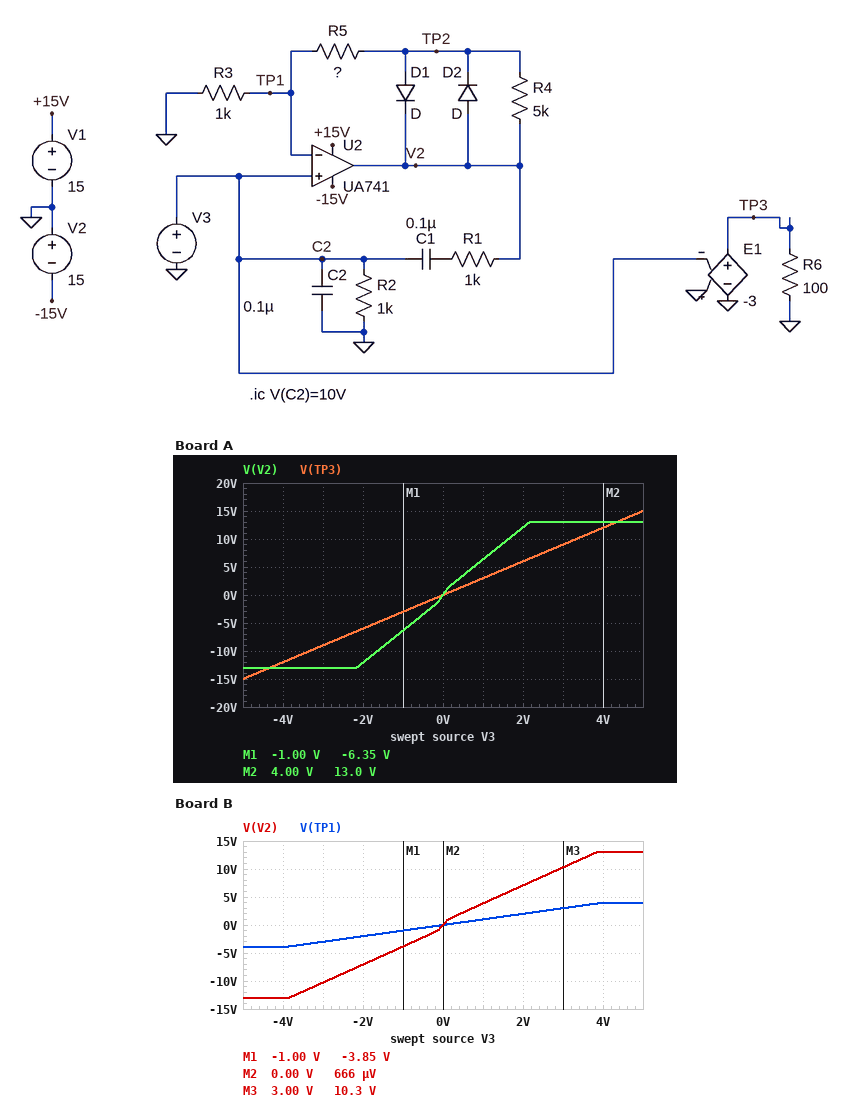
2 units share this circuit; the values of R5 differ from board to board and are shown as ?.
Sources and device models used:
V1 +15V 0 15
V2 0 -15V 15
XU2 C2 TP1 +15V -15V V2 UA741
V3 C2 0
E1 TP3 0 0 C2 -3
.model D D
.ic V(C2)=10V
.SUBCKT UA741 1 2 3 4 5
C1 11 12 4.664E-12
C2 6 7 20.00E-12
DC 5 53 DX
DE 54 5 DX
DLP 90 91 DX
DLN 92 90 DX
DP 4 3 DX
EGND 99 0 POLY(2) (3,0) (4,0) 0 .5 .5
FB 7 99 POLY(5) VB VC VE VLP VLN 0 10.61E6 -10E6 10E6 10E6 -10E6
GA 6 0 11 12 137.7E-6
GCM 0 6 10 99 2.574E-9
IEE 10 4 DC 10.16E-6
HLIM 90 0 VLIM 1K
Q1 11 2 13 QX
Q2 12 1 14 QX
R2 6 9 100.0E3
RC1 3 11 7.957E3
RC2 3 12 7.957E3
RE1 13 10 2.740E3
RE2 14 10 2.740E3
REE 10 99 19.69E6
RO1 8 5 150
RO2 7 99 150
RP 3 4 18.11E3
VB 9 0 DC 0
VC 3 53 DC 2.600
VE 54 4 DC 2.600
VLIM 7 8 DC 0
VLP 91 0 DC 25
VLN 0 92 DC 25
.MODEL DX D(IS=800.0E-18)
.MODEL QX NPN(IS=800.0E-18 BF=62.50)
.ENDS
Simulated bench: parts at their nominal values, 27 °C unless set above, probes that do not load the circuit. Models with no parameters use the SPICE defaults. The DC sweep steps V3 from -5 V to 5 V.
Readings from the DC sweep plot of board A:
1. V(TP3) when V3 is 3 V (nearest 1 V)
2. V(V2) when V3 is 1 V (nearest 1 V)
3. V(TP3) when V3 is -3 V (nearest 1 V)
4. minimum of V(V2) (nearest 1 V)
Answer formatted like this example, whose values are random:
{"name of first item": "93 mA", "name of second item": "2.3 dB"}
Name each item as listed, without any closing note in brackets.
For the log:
{"V(TP3) when V3 is 3 V": "9 V", "V(V2) when V3 is 1 V": "6 V", "V(TP3) when V3 is -3 V": "-9 V", "minimum of V(V2)": "-13 V"}
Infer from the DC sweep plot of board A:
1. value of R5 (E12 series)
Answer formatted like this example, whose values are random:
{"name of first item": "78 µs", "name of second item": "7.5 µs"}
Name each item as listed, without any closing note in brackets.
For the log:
{"value of R5": "4.7 kΩ"}
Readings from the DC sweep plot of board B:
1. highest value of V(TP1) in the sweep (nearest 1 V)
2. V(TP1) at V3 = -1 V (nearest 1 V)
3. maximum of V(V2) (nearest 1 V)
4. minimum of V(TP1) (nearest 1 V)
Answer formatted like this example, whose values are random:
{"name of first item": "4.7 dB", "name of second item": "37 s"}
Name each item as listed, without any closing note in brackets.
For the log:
{"highest value of V(TP1) in the sweep": "4 V", "V(TP1) at V3 = -1 V": "-1 V", "maximum of V(V2)": "13 V", "minimum of V(TP1)": "-4 V"}
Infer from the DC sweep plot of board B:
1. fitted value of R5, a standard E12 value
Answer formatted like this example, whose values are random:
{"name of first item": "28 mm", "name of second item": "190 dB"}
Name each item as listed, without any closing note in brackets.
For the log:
{"fitted value of R5, a standard E12 value": "2.2 kΩ"}
